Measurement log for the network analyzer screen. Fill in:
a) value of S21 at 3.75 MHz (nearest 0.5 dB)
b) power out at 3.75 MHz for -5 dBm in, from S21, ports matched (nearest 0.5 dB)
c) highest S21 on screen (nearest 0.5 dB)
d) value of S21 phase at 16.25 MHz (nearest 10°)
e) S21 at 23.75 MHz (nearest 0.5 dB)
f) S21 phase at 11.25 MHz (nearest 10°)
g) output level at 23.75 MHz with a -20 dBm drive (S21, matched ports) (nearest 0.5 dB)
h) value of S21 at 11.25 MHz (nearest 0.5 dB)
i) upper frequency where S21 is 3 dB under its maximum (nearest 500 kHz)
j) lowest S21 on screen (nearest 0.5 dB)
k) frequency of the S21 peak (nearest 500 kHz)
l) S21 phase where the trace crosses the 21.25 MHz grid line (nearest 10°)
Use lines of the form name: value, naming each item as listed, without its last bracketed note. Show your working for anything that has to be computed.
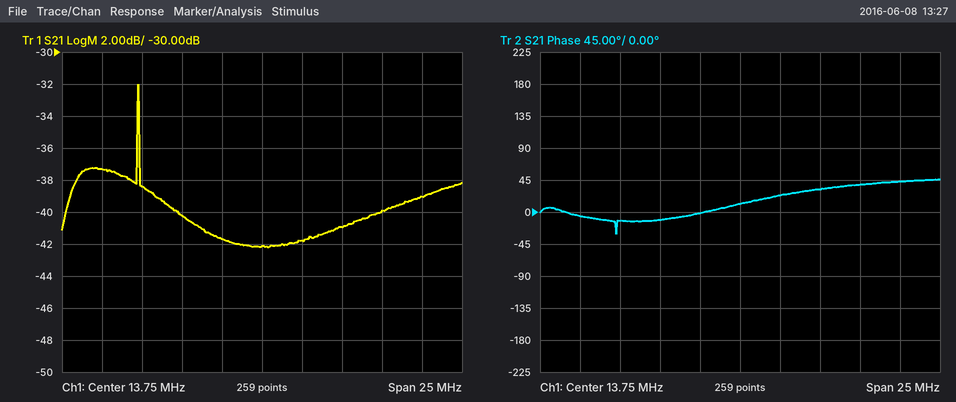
value of S21 at 3.75 MHz: -37.5 dB
power out at 3.75 MHz for -5 dBm in, from S21, ports matched: -5 dBm + (-37.5 dB) = -42.5 dBm
highest S21 on screen: -32.0 dB
value of S21 phase at 16.25 MHz: 20°
S21 at 23.75 MHz: -39.0 dB
S21 phase at 11.25 MHz: 0°
output level at 23.75 MHz with a -20 dBm drive (S21, matched ports): -20 dBm + (-39.0 dB) = -59.0 dBm
value of S21 at 11.25 MHz: -41.5 dB
upper frequency where S21 is 3 dB under its maximum: 6.0 MHz
lowest S21 on screen: -42.0 dB
frequency of the S21 peak: 6.0 MHz
S21 phase where the trace crosses the 21.25 MHz grid line: 40°
